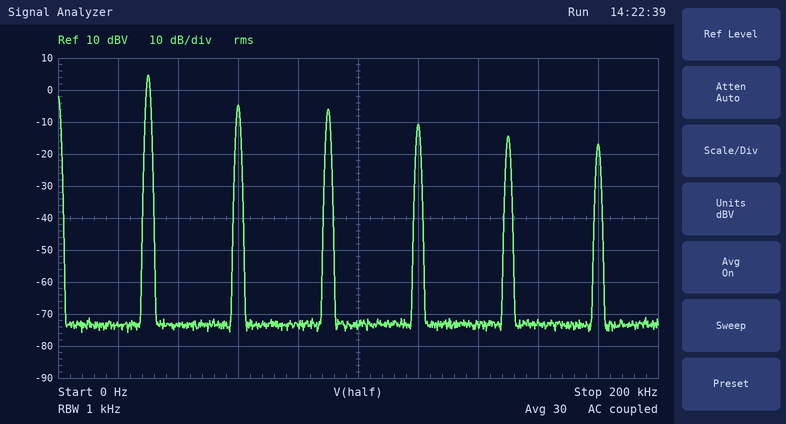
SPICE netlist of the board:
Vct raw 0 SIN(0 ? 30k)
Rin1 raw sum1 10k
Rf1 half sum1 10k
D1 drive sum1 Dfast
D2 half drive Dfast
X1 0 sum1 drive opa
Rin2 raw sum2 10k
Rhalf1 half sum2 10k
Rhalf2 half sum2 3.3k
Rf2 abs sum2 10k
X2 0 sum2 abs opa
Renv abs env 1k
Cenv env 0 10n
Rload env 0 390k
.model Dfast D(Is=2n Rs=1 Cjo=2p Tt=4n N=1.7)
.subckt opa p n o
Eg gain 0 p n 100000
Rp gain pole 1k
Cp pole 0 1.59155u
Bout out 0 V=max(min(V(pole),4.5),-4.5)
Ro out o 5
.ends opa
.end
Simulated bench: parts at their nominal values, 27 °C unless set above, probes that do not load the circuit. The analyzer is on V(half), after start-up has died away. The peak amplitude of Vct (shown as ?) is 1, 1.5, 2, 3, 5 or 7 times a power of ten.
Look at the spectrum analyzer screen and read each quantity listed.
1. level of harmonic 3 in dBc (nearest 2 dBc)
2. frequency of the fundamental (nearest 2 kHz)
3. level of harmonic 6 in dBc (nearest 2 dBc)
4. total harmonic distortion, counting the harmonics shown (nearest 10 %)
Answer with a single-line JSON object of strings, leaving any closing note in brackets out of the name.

{"level of harmonic 3 in dBc": "-10 dBc", "frequency of the fundamental": "30 kHz", "level of harmonic 6 in dBc": "-22 dBc", "total harmonic distortion, counting the harmonics shown": "50 %"}
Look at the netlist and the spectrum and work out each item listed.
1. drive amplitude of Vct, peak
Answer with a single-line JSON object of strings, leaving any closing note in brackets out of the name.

{"drive amplitude of Vct, peak": "5 V"}
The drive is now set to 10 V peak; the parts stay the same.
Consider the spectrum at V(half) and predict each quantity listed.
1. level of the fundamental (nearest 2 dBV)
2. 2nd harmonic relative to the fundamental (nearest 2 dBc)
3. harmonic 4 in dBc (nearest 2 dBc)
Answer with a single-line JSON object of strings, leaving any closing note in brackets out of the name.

{"level of the fundamental": "2 dBV", "2nd harmonic relative to the fundamental": "-8 dBc", "harmonic 4 in dBc": "-10 dBc"}
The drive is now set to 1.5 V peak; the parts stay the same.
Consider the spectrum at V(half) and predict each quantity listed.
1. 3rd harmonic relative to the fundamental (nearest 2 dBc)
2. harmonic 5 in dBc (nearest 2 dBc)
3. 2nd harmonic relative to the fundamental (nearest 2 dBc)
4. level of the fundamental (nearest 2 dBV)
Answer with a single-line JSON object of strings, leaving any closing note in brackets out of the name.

{"3rd harmonic relative to the fundamental": "-48 dBc", "harmonic 5 in dBc": "-50 dBc", "2nd harmonic relative to the fundamental": "-8 dBc", "level of the fundamental": "-6 dBV"}
